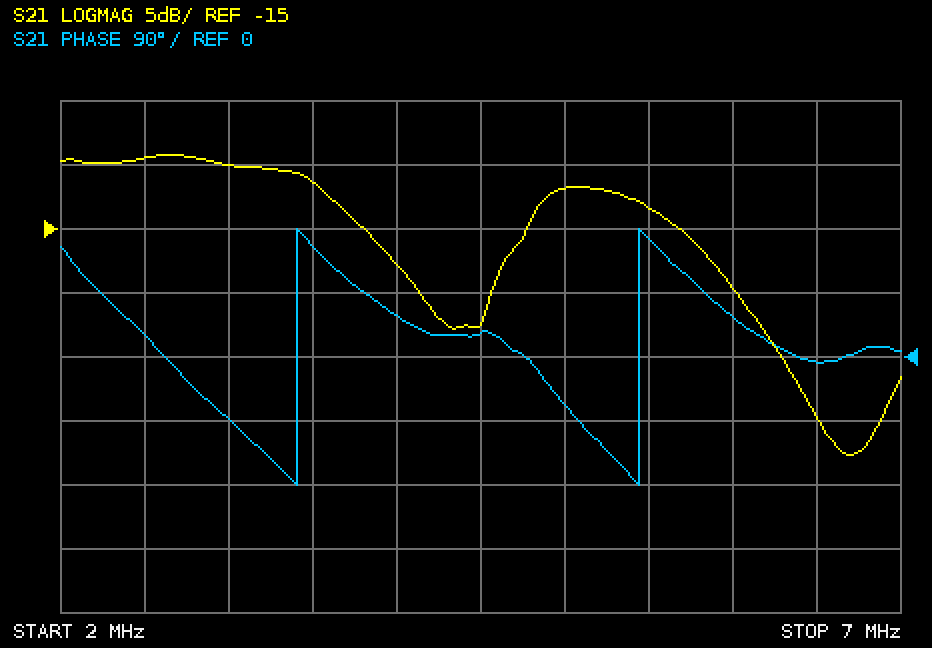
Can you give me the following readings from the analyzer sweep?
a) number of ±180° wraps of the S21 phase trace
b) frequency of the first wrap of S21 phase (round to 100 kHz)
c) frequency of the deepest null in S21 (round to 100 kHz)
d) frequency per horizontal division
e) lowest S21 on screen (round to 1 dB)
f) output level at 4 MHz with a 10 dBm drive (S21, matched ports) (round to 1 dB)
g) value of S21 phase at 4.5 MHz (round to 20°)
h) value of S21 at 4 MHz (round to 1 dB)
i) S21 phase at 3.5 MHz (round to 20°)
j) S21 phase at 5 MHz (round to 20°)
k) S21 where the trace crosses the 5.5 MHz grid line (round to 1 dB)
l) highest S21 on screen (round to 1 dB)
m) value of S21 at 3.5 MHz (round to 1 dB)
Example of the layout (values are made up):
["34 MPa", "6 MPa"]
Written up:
["2", "3.4 MHz", "6.7 MHz", "500 kHz", "-33 dB", "-8 dBm", "40°", "-18 dB", "160°", "-60°", "-13 dB", "-9 dB", "-11 dB"]
